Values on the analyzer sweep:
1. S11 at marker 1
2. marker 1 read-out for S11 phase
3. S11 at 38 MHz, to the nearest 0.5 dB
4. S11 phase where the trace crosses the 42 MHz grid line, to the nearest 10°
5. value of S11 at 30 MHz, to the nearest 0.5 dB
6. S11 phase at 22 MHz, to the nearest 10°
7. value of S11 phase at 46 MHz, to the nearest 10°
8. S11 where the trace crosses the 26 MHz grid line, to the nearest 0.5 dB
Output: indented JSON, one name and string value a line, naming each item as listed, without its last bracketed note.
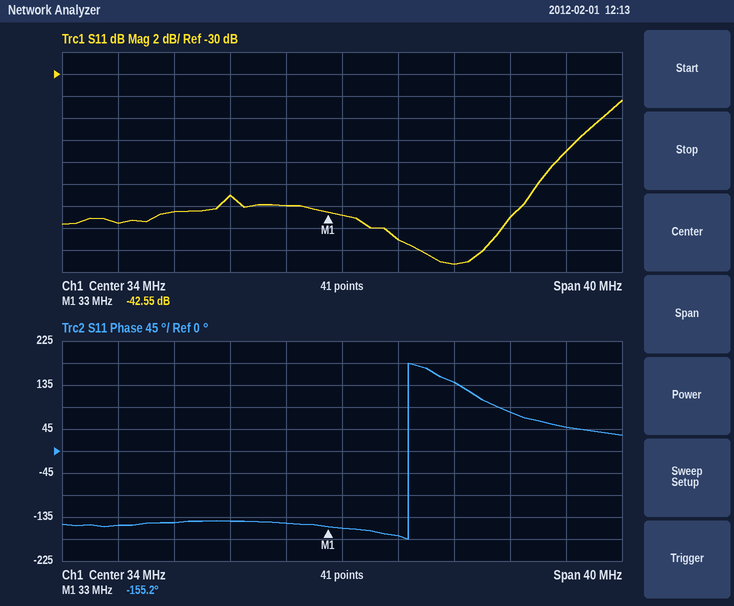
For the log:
{
  "S11 at marker 1": "-42.55 dB",
  "marker 1 read-out for S11 phase": "-155.2°",
  "S11 at 38 MHz, to the nearest 0.5 dB": "-45.0 dB",
  "S11 phase where the trace crosses the 42 MHz grid line, to the nearest 10°": "140°",
  "value of S11 at 30 MHz, to the nearest 0.5 dB": "-42.0 dB",
  "S11 phase at 22 MHz, to the nearest 10°": "-150°",
  "value of S11 phase at 46 MHz, to the nearest 10°": "80°",
  "S11 where the trace crosses the 26 MHz grid line, to the nearest 0.5 dB": "-41.0 dB"
}
